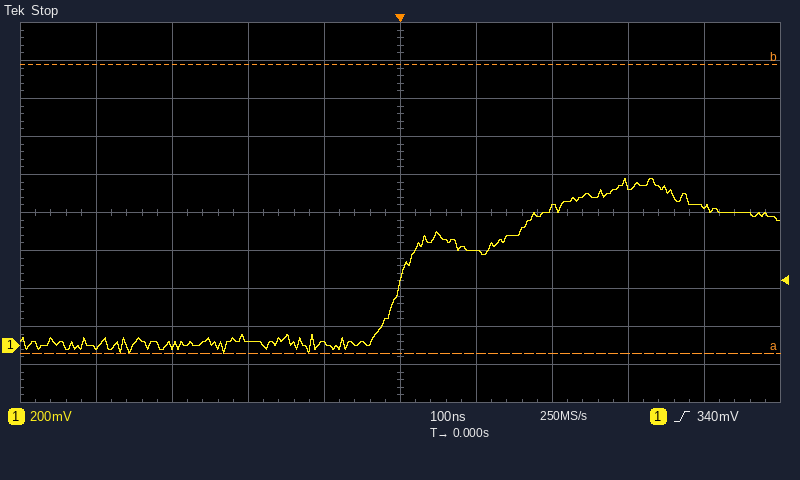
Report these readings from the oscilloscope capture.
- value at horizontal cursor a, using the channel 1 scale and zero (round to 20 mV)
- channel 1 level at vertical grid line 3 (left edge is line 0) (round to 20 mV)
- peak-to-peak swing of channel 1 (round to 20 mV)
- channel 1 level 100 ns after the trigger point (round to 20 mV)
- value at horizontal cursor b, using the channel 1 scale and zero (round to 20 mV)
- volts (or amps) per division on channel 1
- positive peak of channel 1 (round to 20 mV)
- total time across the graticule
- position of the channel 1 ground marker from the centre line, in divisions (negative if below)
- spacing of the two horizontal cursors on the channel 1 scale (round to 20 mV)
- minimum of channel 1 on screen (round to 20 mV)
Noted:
-40 mV
20 mV
920 mV
500 mV
1.48 V
200 mV
880 mV
1 µs
-3.5 div
1.52 V
-40 mV
